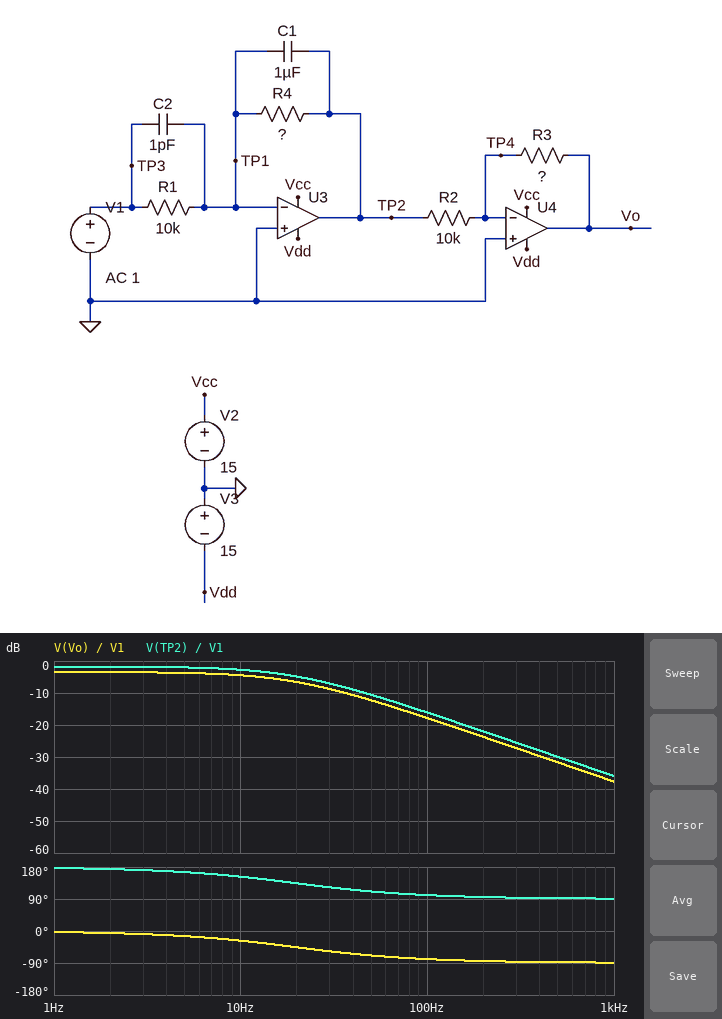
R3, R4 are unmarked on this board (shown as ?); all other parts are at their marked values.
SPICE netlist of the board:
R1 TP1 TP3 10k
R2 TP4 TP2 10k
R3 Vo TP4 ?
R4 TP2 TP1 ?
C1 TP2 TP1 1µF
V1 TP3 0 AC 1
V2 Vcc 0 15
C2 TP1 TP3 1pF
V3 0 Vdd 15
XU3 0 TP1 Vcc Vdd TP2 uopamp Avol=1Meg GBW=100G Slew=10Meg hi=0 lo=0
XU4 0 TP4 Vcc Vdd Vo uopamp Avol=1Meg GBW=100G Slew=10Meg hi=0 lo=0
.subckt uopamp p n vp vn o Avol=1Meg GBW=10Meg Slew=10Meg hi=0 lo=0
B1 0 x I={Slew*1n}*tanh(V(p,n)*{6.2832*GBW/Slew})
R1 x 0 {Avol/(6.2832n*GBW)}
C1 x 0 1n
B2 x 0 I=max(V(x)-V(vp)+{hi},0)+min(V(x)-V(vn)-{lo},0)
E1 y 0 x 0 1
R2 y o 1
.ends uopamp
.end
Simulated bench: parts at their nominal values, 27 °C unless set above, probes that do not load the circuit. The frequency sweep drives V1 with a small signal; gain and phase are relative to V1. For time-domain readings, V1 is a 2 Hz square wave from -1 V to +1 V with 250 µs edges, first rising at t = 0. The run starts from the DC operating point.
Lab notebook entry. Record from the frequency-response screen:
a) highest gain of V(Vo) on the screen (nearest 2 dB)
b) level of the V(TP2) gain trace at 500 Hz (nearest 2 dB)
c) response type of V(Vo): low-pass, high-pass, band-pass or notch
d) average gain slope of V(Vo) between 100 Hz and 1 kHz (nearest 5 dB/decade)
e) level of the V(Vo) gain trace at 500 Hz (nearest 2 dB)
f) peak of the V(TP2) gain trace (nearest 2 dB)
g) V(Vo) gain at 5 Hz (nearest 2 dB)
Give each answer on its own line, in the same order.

-4 dB
-30 dB
low-pass
-20 dB/decade
-32 dB
-2 dB
-4 dB
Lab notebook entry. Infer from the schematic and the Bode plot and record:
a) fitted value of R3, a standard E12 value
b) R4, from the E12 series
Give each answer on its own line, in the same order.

8.2 kΩ
8.2 kΩ
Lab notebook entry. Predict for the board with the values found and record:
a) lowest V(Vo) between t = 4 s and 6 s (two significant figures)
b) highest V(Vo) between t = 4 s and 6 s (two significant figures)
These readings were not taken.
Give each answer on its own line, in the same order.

-670 mV
670 mV
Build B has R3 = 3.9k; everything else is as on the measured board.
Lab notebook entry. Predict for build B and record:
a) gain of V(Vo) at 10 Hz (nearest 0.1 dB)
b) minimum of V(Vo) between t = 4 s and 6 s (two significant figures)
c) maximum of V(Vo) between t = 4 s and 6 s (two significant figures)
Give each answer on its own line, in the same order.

-10.9 dB
-320 mV
320 mV
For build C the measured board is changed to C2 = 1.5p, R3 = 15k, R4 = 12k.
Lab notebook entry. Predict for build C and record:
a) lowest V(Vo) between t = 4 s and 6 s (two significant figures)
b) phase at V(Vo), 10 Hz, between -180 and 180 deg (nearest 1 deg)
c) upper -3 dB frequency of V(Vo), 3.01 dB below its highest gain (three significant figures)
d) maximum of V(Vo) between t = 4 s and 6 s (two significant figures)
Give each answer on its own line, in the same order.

-1.8 V
-37 deg
13.3 Hz
1.8 V
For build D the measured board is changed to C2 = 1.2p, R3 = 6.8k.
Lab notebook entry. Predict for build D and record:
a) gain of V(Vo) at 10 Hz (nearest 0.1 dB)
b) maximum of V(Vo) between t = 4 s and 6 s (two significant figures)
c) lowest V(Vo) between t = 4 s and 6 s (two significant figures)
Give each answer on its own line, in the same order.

-6.1 dB
560 mV
-560 mV
